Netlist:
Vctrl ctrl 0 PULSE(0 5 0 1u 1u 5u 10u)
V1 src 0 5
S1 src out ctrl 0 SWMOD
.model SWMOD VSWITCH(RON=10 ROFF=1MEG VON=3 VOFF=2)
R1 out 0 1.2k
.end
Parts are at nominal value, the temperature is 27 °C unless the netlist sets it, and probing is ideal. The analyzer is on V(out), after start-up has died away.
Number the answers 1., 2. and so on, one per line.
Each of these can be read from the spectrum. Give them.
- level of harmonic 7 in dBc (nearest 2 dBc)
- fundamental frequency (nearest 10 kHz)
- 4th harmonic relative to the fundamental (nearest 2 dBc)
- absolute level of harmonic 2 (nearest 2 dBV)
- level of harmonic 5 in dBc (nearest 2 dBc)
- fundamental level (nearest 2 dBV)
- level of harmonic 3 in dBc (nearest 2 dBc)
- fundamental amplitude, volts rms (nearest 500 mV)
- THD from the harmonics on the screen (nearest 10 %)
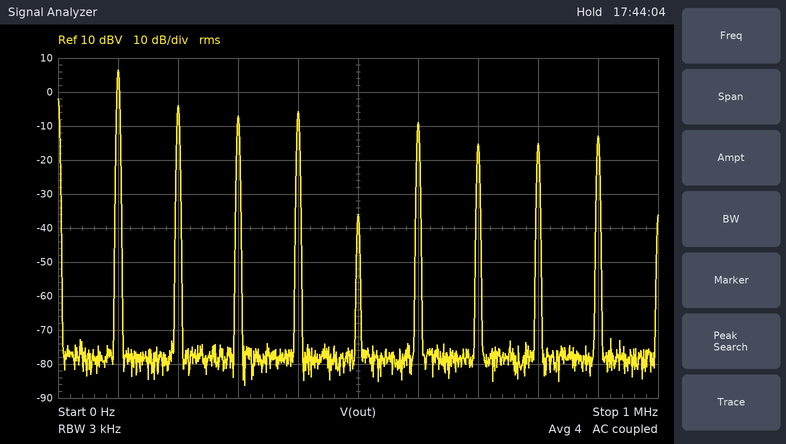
1. -22 dBc
2. 100 kHz
3. -12 dBc
4. -4 dBV
5. -42 dBc
6. 6 dBV
7. -14 dBc
8. 2.0 V
9. 50 %
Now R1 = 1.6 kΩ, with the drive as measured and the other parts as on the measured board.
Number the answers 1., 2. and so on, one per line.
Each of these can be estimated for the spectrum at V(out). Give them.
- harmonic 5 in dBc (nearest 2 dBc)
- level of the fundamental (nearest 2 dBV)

1. -46 dBc
2. 6 dBV
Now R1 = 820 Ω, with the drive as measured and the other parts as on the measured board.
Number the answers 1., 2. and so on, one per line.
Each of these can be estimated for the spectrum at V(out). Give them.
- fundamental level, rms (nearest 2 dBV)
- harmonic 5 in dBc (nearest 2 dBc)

1. 6 dBV
2. -40 dBc
